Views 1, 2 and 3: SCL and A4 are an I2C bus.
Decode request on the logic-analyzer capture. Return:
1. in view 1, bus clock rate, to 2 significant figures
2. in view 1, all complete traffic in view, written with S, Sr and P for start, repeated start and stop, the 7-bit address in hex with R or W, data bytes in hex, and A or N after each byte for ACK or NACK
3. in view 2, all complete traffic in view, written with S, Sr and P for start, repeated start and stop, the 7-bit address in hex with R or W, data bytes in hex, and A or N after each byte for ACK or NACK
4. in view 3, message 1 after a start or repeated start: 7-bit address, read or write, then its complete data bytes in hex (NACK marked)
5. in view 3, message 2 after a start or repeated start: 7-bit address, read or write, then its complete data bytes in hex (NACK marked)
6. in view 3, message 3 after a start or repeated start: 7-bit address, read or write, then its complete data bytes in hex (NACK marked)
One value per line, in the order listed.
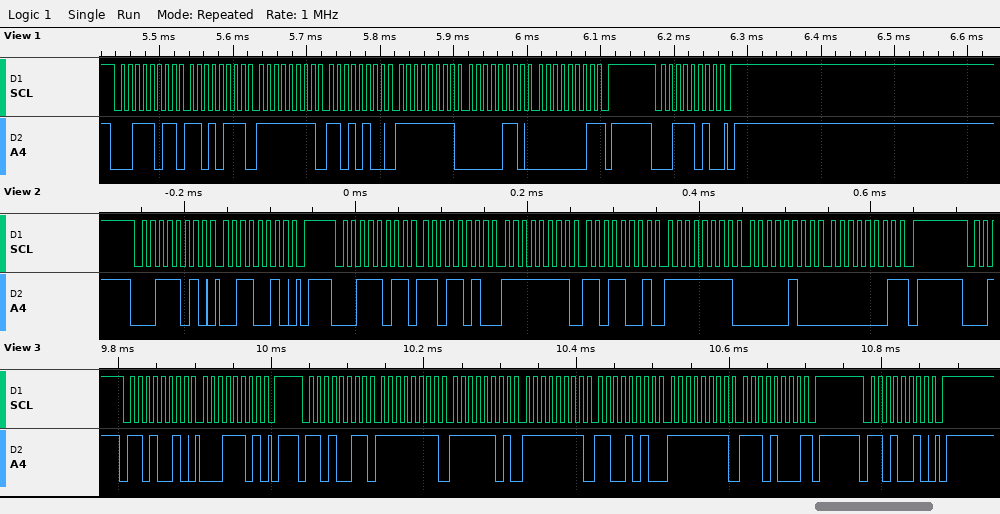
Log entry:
100 kHz
S 1DR A D7 A FF A D4 A FF A 06 A 01 N P S 1DW A P
S 1DW A 32 A P S 1DR A DA A FF A D9 A FF A 04 A 01 N P
0x69 write: 1D
0x69 read: FF FD FF CA FF E8 NACK
0x69 write
